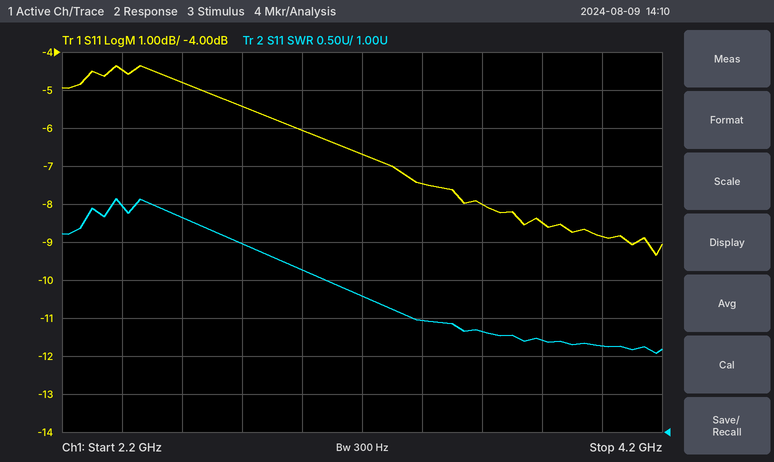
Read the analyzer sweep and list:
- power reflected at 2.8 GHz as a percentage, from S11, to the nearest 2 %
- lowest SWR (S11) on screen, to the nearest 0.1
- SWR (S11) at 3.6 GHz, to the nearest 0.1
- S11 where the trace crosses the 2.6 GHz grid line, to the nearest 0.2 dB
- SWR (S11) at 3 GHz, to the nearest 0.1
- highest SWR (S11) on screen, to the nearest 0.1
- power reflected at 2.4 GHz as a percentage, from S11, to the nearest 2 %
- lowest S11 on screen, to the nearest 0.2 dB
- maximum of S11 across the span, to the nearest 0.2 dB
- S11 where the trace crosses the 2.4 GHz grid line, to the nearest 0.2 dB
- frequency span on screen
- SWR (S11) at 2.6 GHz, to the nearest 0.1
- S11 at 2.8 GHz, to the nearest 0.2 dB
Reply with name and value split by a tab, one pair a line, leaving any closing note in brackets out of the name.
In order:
power reflected at 2.8 GHz as a percentage, from S11, to the nearest 2 %	28 %
lowest SWR (S11) on screen, to the nearest 0.1	2.0
SWR (S11) at 3.6 GHz, to the nearest 0.1	2.3
S11 where the trace crosses the 2.6 GHz grid line, to the nearest 0.2 dB	-4.8 dB
SWR (S11) at 3 GHz, to the nearest 0.1	3.1
highest SWR (S11) on screen, to the nearest 0.1	4.1
power reflected at 2.4 GHz as a percentage, from S11, to the nearest 2 %	36 %
lowest S11 on screen, to the nearest 0.2 dB	-9.4 dB
maximum of S11 across the span, to the nearest 0.2 dB	-4.4 dB
S11 where the trace crosses the 2.4 GHz grid line, to the nearest 0.2 dB	-4.4 dB
frequency span on screen	2 GHz
SWR (S11) at 2.6 GHz, to the nearest 0.1	3.8
S11 at 2.8 GHz, to the nearest 0.2 dB	-5.4 dB
